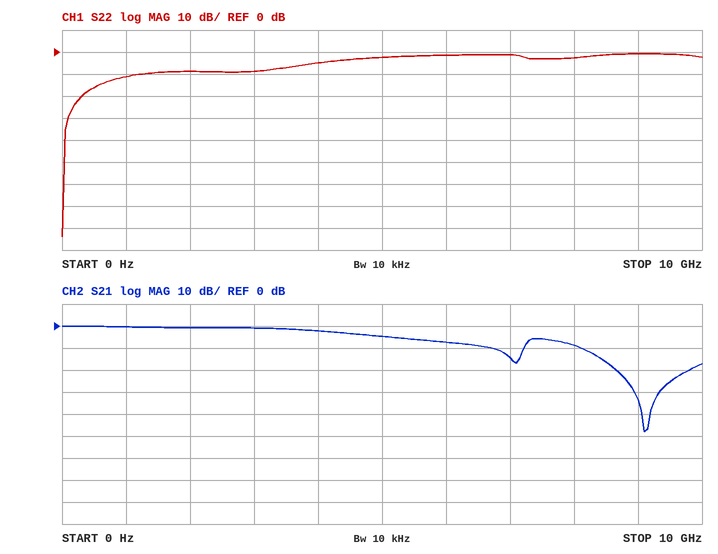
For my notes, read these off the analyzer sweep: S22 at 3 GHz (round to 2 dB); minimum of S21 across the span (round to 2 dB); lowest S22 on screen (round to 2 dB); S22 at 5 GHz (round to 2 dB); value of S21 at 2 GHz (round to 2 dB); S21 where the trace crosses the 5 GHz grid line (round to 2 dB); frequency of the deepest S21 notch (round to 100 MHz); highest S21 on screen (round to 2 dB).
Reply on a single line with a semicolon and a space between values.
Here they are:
-8 dB; -48 dB; -84 dB; -2 dB; 0 dB; -4 dB; 9.1 GHz; 0 dB
